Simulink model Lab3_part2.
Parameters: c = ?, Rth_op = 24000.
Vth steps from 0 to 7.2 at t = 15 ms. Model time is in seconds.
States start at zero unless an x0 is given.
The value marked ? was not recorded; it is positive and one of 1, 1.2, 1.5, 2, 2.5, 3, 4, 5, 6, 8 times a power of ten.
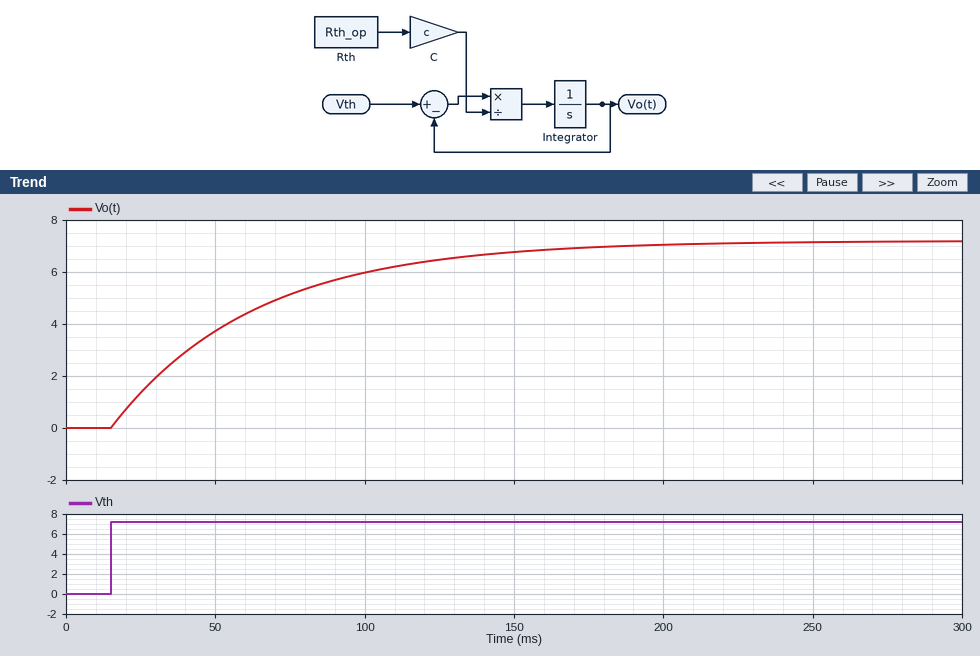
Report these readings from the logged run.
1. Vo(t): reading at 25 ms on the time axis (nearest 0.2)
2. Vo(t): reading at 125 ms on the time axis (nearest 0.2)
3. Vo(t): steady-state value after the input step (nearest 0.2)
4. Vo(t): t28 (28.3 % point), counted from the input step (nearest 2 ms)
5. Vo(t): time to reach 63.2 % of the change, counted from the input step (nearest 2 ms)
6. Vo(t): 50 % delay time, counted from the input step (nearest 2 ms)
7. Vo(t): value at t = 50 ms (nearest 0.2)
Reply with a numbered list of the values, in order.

1. 1.4
2. 6.4
3. 7.2
4. 16 ms
5. 48 ms
6. 34 ms
7. 3.8
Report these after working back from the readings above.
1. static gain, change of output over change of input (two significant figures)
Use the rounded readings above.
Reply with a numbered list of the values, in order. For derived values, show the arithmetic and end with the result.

1. (7.2 - 0) / (7.2 - 0) = 1.0
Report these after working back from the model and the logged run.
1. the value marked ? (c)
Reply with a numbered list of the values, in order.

1. 2e-06
